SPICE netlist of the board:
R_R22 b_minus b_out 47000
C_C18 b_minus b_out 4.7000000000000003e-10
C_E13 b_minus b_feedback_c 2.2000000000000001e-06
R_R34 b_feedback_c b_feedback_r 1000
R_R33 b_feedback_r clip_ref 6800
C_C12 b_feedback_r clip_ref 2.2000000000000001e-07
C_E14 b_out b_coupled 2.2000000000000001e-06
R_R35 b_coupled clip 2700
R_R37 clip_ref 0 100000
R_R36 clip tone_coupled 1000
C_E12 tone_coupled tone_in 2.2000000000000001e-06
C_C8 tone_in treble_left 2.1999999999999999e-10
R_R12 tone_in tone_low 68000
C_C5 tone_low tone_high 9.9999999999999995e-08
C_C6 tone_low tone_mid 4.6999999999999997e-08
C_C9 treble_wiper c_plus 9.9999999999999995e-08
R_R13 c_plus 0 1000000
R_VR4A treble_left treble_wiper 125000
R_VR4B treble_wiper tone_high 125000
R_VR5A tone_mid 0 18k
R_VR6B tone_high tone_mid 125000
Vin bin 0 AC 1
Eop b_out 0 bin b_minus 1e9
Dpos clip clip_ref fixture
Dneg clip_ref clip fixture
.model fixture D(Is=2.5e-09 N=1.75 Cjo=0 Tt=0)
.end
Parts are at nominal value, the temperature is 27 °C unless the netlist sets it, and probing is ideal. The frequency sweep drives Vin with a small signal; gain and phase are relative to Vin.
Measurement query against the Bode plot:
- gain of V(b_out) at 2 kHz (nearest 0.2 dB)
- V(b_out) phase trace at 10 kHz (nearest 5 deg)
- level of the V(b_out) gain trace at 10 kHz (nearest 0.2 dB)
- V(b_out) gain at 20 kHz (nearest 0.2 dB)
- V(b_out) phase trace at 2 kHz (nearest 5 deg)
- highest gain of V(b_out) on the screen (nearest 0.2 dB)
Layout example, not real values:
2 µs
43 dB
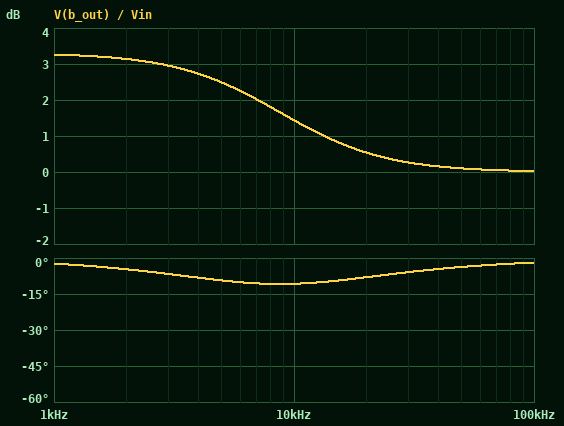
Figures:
3.2 dB
-10 deg
1.4 dB
0.6 dB
-5 deg
3.2 dB
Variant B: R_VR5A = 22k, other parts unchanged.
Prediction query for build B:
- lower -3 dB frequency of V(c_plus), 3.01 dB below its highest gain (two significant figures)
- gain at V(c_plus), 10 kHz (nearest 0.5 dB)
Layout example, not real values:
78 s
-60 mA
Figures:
7.0 Hz
-3.5 dB
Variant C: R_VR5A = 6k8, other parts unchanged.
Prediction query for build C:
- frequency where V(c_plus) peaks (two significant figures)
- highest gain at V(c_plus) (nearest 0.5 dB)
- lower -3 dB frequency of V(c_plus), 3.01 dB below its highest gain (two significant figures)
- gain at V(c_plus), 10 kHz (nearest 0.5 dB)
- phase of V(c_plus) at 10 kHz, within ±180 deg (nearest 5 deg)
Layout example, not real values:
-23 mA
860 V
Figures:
27 Hz
-3.5 dB
7.5 Hz
-5.0 dB
5 deg
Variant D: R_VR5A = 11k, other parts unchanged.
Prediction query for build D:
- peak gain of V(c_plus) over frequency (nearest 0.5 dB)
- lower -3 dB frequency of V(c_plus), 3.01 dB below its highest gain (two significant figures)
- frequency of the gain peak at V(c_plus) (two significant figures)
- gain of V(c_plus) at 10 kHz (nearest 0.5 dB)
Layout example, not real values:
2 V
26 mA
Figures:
-3.5 dB
7.3 Hz
26 Hz
-4.5 dB
